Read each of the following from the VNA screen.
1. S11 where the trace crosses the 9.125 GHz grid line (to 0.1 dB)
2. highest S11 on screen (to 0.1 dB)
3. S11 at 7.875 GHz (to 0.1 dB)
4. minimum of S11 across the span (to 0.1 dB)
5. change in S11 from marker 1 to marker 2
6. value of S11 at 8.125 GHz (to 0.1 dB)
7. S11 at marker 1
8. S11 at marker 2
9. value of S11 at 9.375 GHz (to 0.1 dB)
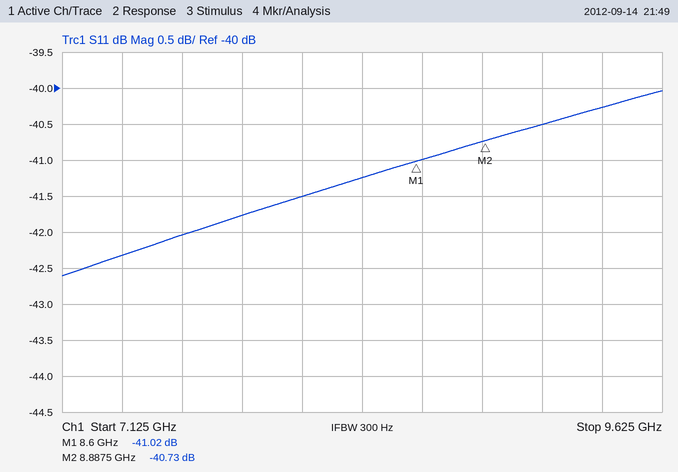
-40.5 dB
-40.0 dB
-41.8 dB
-42.6 dB
0.29 dB
-41.5 dB
-41.02 dB
-40.73 dB
-40.3 dB
